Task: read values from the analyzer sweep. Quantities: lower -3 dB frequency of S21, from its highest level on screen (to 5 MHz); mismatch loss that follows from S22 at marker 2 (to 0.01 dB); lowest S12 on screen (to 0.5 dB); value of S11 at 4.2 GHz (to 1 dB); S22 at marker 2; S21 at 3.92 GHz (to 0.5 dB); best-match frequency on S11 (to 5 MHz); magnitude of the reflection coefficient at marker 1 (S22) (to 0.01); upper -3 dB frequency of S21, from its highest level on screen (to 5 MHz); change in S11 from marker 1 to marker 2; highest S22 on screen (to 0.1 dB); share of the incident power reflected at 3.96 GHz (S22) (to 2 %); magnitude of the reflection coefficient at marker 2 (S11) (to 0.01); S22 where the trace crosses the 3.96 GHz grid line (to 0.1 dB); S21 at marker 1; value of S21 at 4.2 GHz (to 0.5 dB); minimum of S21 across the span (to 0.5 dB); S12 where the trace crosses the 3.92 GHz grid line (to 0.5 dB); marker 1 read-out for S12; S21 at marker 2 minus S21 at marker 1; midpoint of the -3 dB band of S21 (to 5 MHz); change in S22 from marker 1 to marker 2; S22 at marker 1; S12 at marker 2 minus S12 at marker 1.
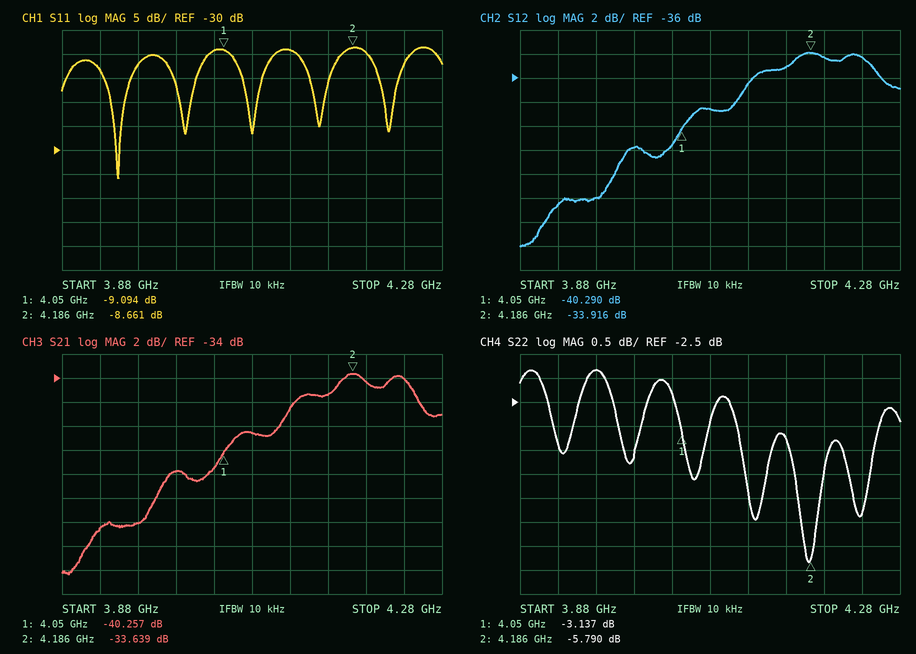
4.120 GHz
1.33 dB
-50.0 dB
-10 dB
-5.790 dB
-46.5 dB
3.940 GHz
0.70
4.260 GHz
0.433 dB
-1.8 dB
66 %
0.37
-1.8 dB
-40.257 dB
-34.5 dB
-50.5 dB
-46.5 dB
-40.290 dB
6.618 dB
4.190 GHz
-2.653 dB
-3.137 dB
6.374 dB
